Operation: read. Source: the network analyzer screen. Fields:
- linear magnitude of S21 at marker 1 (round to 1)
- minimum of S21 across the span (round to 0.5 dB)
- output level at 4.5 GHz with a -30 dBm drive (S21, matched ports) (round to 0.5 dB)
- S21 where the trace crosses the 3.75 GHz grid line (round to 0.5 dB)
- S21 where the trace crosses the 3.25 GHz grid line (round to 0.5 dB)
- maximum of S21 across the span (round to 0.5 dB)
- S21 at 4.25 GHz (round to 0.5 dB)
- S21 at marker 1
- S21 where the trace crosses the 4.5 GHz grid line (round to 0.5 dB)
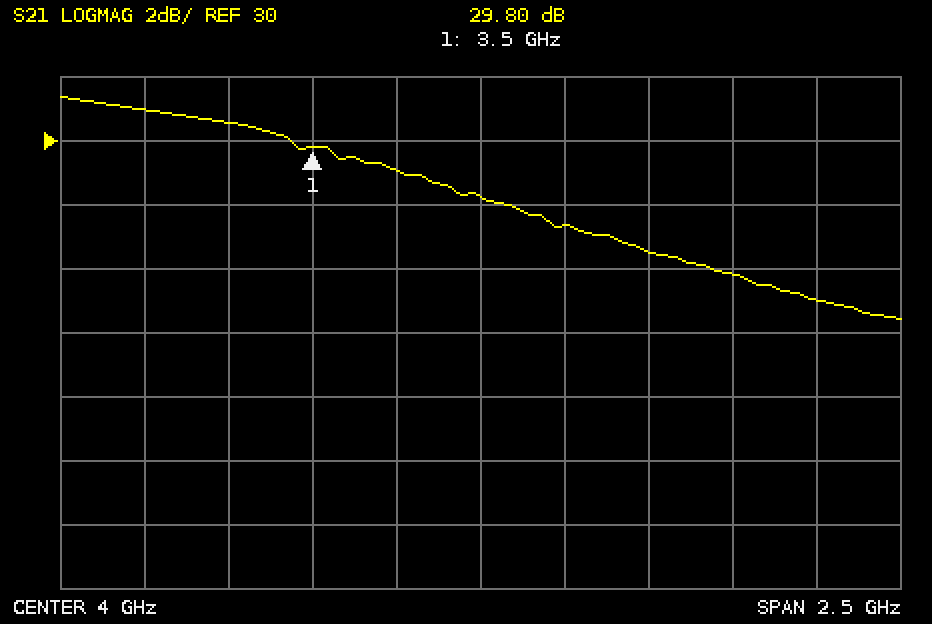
31
24.5 dB
-3.5 dBm
29.0 dB
30.5 dB
31.5 dB
27.5 dB
29.80 dB
26.5 dB
